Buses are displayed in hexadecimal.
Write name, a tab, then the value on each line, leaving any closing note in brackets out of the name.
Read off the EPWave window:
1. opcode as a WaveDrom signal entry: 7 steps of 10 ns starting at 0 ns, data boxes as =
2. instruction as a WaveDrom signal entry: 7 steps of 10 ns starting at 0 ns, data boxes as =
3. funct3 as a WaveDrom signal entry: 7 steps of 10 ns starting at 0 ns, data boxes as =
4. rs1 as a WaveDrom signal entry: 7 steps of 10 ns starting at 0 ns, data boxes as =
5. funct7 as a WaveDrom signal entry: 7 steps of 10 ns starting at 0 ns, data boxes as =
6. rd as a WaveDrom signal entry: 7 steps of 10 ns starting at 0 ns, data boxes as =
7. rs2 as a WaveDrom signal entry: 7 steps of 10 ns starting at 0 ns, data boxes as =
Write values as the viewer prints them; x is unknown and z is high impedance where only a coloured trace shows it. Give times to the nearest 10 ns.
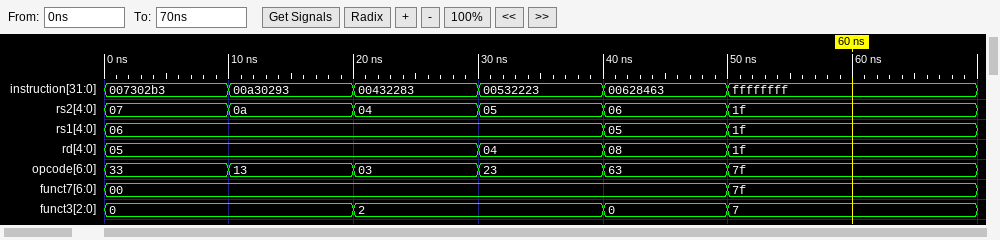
opcode as a WaveDrom signal entry: 7 steps of 10 ns starting at 0 ns, data boxes as =	{name: 'opcode', wave: '======.', data: '33 13 03 23 63 7f'}
instruction as a WaveDrom signal entry: 7 steps of 10 ns starting at 0 ns, data boxes as =	{name: 'instruction', wave: '======.', data: '007302b3 00a30293 00432283 00532223 00628463 ffffffff'}
funct3 as a WaveDrom signal entry: 7 steps of 10 ns starting at 0 ns, data boxes as =	{name: 'funct3', wave: '=.=.==.', data: '0 2 0 7'}
rs1 as a WaveDrom signal entry: 7 steps of 10 ns starting at 0 ns, data boxes as =	{name: 'rs1', wave: '=...==.', data: '06 05 1f'}
funct7 as a WaveDrom signal entry: 7 steps of 10 ns starting at 0 ns, data boxes as =	{name: 'funct7', wave: '=....=.', data: '00 7f'}
rd as a WaveDrom signal entry: 7 steps of 10 ns starting at 0 ns, data boxes as =	{name: 'rd', wave: '=..===.', data: '05 04 08 1f'}
rs2 as a WaveDrom signal entry: 7 steps of 10 ns starting at 0 ns, data boxes as =	{name: 'rs2', wave: '======.', data: '07 0a 04 05 06 1f'}
